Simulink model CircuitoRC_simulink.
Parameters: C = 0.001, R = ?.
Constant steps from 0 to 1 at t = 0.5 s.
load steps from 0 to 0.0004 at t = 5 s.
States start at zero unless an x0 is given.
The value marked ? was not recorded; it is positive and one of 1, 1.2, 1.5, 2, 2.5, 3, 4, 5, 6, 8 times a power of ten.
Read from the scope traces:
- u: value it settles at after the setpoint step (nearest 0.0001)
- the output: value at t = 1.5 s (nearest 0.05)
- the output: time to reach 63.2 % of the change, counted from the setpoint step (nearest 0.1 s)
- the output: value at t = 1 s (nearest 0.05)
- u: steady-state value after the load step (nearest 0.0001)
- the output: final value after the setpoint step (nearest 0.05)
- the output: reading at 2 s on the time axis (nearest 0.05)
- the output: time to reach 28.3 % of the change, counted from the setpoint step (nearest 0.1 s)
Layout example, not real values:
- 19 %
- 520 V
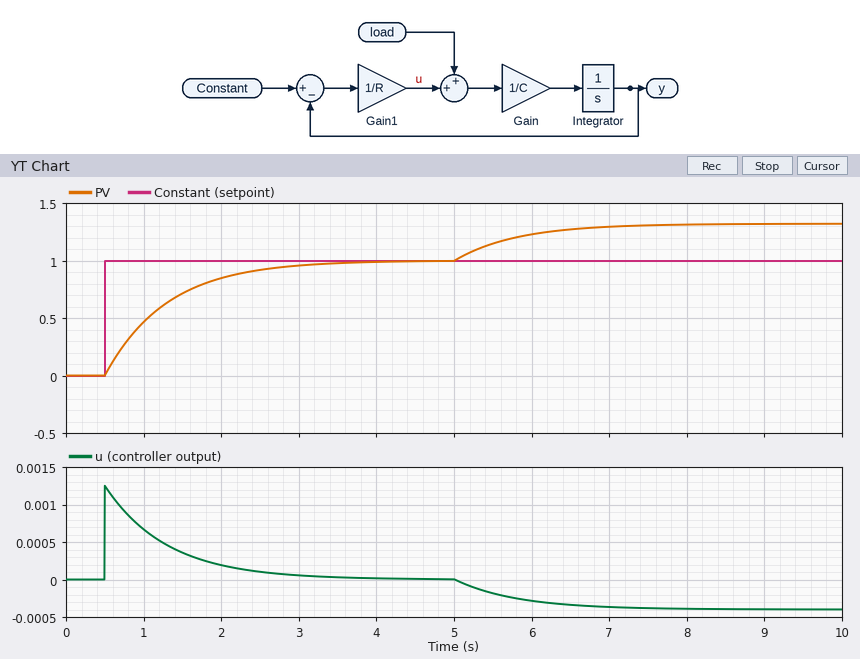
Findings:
- 0.0000
- 0.70
- 0.8 s
- 0.45
- -0.0004
- 1.00
- 0.85
- 0.3 s
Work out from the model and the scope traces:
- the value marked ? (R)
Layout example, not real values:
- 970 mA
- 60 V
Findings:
- 800
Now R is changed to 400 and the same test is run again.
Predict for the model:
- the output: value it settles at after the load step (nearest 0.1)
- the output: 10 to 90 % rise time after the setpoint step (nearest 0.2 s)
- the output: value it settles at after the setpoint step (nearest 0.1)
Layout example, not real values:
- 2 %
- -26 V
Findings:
- 1.2
- 0.8 s
- 1.0
